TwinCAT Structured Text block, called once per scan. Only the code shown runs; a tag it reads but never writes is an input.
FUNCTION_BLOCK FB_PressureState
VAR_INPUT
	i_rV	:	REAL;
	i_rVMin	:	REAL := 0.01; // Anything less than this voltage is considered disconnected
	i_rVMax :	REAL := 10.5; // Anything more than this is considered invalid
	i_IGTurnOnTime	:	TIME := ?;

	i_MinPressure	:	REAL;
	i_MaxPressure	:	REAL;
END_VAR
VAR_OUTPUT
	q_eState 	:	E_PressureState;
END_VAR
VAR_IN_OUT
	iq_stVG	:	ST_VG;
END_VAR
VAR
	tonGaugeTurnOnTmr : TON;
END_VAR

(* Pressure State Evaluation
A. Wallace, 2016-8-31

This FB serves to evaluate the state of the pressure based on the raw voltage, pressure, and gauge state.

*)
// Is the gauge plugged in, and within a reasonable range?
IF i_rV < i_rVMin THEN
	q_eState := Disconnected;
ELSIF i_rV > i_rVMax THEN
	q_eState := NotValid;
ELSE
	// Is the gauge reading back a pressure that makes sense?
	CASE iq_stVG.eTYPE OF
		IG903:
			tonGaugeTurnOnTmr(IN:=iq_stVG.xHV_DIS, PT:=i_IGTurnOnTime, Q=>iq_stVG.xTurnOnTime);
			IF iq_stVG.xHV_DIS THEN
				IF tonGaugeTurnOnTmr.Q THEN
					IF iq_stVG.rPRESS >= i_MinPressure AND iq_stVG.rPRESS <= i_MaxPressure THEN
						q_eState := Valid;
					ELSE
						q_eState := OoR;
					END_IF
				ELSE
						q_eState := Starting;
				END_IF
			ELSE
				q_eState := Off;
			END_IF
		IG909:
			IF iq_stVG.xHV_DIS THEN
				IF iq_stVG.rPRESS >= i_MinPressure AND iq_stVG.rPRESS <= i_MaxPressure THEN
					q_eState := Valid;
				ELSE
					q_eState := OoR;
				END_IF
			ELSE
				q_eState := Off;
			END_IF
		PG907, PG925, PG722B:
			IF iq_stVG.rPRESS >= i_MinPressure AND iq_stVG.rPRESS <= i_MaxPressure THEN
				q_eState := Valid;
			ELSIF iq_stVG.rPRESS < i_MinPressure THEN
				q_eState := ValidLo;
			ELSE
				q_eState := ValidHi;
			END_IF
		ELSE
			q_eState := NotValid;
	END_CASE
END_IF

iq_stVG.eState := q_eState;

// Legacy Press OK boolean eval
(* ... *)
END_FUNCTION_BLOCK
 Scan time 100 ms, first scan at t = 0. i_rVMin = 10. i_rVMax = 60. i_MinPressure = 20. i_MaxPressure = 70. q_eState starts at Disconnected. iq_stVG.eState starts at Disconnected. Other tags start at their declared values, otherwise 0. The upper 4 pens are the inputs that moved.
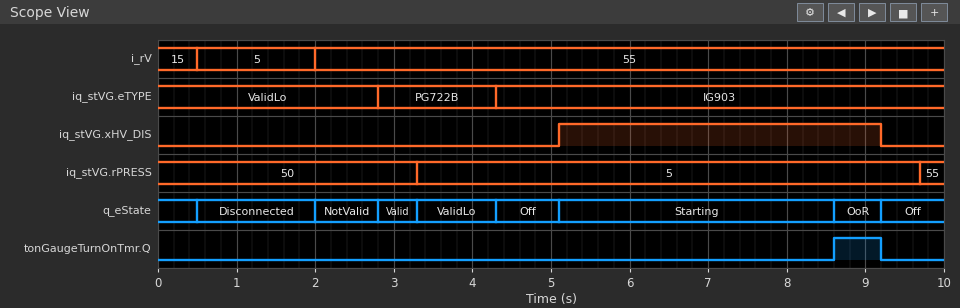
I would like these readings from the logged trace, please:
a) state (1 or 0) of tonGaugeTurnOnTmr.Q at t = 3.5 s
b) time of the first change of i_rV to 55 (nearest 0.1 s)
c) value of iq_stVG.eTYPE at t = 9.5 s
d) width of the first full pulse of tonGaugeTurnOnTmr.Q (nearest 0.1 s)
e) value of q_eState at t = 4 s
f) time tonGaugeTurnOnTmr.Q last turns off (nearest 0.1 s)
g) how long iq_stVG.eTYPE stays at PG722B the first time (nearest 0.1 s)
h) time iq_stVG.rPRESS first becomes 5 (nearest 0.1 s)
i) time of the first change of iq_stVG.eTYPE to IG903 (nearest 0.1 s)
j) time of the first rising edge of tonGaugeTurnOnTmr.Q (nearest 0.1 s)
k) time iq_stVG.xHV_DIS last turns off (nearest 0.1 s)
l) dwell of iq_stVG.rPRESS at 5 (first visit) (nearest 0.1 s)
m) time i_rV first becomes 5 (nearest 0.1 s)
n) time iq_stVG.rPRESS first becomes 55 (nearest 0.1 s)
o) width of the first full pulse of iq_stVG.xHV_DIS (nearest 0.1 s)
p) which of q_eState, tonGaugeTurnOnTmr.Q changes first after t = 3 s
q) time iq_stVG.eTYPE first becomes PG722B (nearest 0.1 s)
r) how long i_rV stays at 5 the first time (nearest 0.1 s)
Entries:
0
2.0 s
IG903
0.6 s
ValidLo
9.2 s
1.5 s
3.3 s
4.3 s
8.6 s
9.2 s
6.4 s
0.5 s
9.7 s
4.1 s
q_eState
2.8 s
1.5 s
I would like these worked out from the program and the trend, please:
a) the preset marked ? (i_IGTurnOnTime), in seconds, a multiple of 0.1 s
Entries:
3.5 s
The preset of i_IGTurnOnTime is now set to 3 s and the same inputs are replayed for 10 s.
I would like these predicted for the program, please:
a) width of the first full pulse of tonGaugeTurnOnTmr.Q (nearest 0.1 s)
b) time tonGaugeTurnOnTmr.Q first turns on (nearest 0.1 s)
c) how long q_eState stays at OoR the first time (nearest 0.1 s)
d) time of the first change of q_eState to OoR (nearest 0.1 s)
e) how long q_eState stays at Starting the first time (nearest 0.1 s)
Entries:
1.1 s
8.1 s
1.1 s
8.1 s
3.0 s
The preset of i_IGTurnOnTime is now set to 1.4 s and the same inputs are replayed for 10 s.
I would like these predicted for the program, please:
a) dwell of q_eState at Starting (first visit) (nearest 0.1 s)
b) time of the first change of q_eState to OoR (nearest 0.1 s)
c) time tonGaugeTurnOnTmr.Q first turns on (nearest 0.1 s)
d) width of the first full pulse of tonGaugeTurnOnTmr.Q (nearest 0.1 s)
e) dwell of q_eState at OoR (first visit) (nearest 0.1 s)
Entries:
1.4 s
6.5 s
6.5 s
2.7 s
2.7 s
